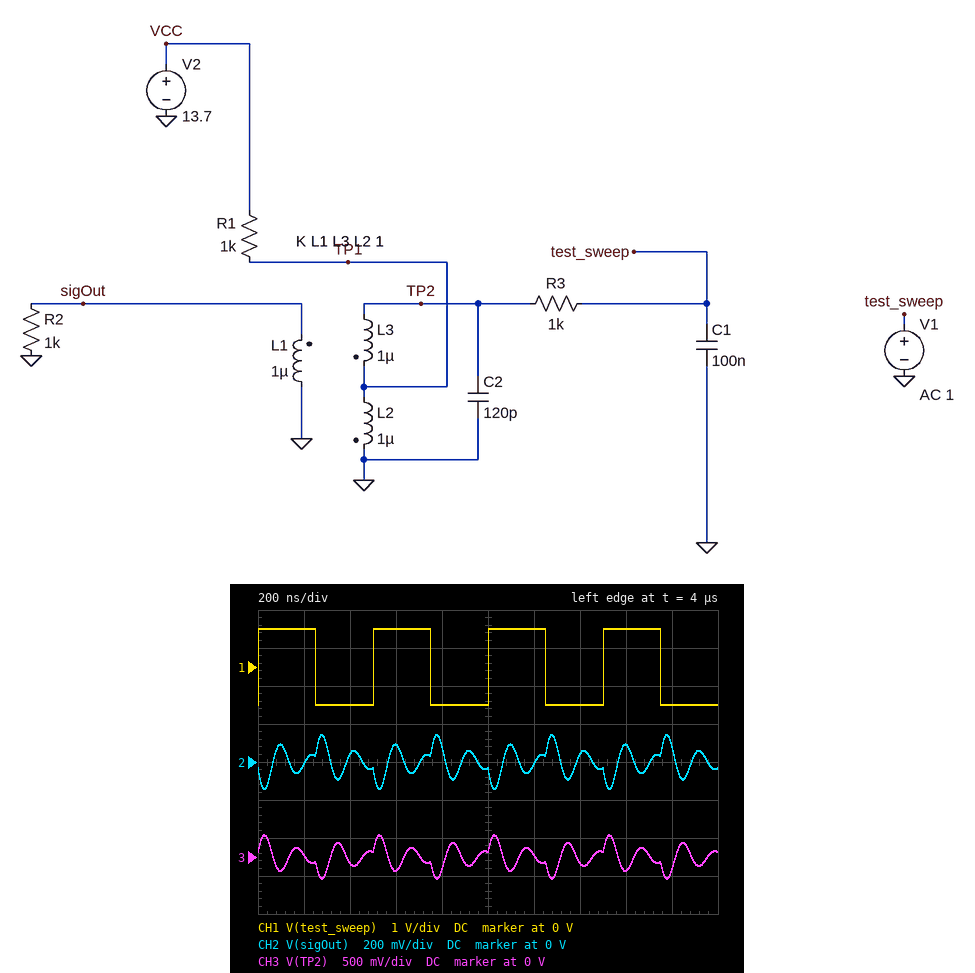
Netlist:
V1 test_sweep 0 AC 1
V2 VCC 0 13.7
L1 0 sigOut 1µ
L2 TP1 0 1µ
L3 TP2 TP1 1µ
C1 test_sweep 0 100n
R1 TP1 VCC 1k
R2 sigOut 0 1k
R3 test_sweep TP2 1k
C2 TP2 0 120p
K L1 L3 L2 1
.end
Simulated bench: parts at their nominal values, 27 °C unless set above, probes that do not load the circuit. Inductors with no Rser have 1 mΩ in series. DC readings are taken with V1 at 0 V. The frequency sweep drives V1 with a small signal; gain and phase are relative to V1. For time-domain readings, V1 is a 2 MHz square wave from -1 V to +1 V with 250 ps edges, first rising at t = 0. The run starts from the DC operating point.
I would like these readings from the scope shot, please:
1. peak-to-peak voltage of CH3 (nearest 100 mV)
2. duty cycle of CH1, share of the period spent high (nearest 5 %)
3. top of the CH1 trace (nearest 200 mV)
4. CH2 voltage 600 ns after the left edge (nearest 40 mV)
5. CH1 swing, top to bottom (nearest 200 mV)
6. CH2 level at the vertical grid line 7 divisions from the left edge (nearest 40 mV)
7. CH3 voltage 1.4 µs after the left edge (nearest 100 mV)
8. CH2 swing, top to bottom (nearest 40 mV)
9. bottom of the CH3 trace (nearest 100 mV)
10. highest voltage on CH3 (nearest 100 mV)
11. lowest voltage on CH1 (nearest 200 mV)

600 mV
50 %
1.0 V
80 mV
2.0 V
40 mV
-100 mV
280 mV
-300 mV
300 mV
-1.0 V
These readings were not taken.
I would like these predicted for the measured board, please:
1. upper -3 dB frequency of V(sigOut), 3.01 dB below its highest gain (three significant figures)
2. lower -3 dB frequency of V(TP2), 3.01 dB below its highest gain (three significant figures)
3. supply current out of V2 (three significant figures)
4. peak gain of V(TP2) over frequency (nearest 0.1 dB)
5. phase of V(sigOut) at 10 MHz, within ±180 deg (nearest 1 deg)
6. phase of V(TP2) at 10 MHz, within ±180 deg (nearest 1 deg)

8.33 MHz
6.34 MHz
13.7 mA
-3.5 dB
113 deg
-67 deg
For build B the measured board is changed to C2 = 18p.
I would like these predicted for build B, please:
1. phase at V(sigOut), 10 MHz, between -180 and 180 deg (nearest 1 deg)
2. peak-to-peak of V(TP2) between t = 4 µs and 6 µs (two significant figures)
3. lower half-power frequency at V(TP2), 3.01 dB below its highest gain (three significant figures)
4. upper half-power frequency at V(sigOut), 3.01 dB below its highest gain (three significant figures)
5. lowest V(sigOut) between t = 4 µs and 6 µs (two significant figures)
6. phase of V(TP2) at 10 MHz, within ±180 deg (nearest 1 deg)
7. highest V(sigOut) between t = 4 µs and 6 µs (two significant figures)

-118 deg
1.2 V
13.3 MHz
26.5 MHz
-300 mV
62 deg
300 mV
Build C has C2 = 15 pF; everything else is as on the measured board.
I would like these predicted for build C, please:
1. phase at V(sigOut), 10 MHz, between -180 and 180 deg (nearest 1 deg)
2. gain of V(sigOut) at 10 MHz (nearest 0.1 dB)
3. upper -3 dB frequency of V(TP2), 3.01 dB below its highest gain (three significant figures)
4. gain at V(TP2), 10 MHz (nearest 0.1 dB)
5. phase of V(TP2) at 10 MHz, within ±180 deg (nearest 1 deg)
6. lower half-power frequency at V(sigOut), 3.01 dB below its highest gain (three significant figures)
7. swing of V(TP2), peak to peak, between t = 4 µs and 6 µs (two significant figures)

-116 deg
-16.6 dB
30.0 MHz
-10.6 dB
64 deg
14.1 MHz
1.3 V
